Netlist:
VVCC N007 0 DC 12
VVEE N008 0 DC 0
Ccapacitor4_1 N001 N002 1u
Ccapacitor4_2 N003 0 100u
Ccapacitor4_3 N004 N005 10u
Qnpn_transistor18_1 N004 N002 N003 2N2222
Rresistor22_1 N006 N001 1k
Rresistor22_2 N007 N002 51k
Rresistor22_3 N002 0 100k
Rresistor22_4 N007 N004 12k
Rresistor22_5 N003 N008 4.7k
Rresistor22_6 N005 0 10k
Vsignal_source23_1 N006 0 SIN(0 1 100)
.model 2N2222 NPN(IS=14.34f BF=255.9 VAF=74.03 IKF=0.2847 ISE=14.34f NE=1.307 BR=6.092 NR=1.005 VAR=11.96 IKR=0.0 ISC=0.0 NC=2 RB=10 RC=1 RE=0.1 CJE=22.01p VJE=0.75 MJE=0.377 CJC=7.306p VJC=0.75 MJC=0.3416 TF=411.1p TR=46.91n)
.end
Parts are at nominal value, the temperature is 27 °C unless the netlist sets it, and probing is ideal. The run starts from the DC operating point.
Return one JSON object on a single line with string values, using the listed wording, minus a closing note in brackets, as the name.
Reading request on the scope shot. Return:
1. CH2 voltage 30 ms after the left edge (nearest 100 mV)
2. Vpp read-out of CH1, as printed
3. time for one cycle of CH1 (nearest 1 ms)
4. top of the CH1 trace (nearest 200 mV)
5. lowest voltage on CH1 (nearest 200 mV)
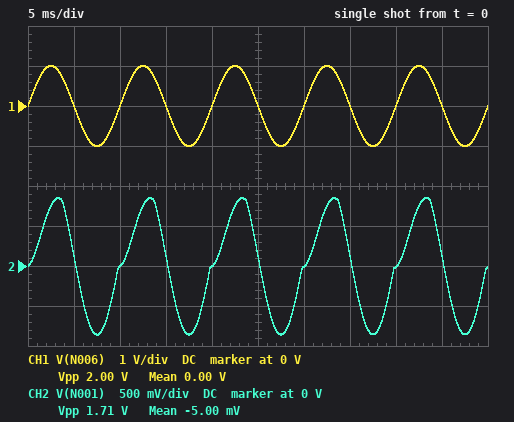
{"CH2 voltage 30 ms after the left edge": "0 V", "Vpp read-out of CH1, as printed": "2.00 V", "time for one cycle of CH1": "10 ms", "top of the CH1 trace": "1.0 V", "lowest voltage on CH1": "-1.0 V"}
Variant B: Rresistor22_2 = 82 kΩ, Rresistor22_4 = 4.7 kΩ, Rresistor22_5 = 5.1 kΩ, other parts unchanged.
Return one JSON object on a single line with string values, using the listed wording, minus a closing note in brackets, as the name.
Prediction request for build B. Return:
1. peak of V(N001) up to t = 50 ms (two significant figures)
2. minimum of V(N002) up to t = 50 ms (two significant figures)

{"peak of V(N001) up to t = 50 ms": "890 mV", "minimum of V(N002) up to t = 50 ms": "4.3 V"}
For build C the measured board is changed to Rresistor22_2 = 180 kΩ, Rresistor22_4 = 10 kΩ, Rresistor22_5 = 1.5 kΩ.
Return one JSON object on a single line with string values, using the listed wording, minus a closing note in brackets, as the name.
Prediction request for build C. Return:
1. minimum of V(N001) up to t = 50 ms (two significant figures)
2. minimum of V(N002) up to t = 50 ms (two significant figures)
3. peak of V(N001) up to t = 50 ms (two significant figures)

{"minimum of V(N001) up to t = 50 ms": "-940 mV", "minimum of V(N002) up to t = 50 ms": "410 mV", "peak of V(N001) up to t = 50 ms": "880 mV"}
